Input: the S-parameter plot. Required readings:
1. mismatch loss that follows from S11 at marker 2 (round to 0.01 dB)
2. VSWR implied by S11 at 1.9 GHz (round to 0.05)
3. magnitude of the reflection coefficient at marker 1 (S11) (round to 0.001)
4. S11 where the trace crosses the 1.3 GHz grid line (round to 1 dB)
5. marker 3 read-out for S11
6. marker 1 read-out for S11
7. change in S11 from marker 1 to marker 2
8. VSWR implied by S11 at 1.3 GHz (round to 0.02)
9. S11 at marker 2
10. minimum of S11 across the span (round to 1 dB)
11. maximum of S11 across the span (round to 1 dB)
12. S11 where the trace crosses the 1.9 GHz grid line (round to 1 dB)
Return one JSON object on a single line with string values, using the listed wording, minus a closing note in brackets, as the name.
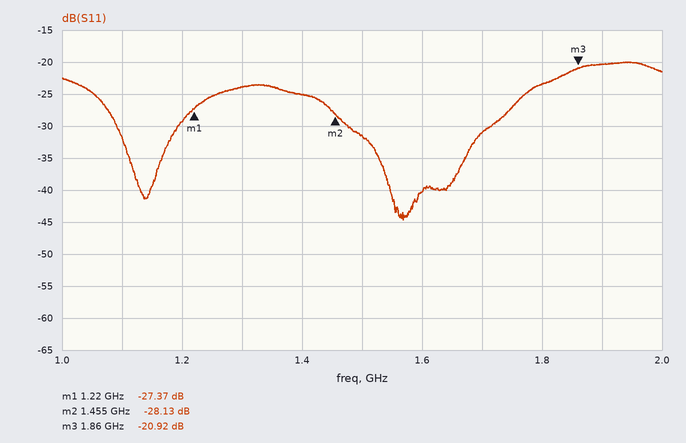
{"mismatch loss that follows from S11 at marker 2": "0.01 dB", "VSWR implied by S11 at 1.9 GHz": "1.20", "magnitude of the reflection coefficient at marker 1 (S11)": "0.043", "S11 where the trace crosses the 1.3 GHz grid line": "-24 dB", "marker 3 read-out for S11": "-20.92 dB", "marker 1 read-out for S11": "-27.37 dB", "change in S11 from marker 1 to marker 2": "-0.76 dB", "VSWR implied by S11 at 1.3 GHz": "1.14", "S11 at marker 2": "-28.13 dB", "minimum of S11 across the span": "-45 dB", "maximum of S11 across the span": "-20 dB", "S11 where the trace crosses the 1.9 GHz grid line": "-20 dB"}
